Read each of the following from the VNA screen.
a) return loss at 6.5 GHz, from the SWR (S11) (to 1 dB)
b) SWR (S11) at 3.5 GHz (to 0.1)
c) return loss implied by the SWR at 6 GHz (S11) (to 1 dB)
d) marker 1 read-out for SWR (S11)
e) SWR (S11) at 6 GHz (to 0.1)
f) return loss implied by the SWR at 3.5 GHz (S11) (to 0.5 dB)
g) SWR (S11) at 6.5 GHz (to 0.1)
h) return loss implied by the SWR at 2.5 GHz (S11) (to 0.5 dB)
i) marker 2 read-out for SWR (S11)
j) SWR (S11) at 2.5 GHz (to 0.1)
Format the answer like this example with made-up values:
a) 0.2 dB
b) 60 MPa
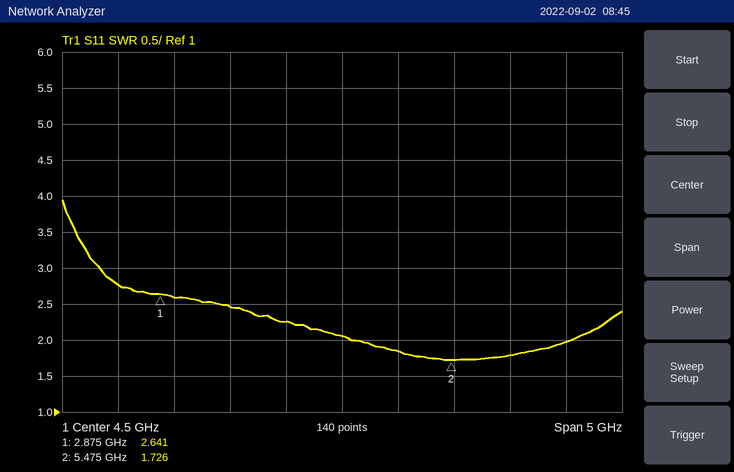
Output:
a) 10 dB
b) 2.5
c) 11 dB
d) 2.641
e) 1.8
f) 7.5 dB
g) 2.0
h) 6.5 dB
i) 1.726
j) 2.8
